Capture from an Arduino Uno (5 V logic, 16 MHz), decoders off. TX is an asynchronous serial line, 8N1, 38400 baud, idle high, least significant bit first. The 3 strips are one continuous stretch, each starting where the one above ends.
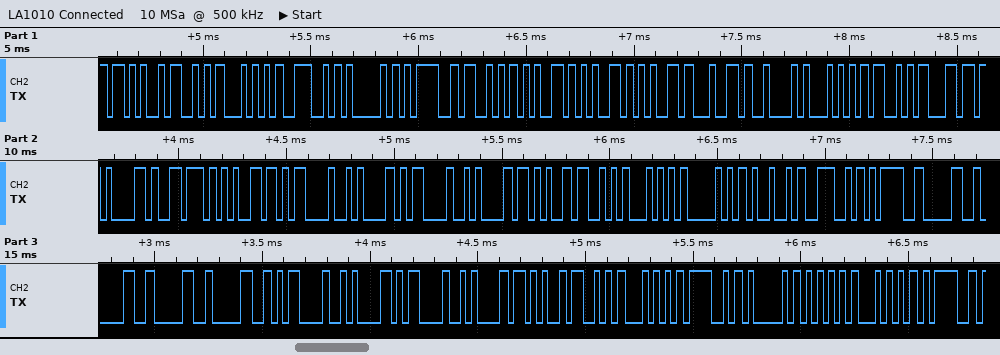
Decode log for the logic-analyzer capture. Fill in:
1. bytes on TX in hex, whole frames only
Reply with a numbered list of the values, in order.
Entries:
1. 0x2B 0x53 0x54 0x4E 0x41 0x3D 0x53 0x65 0x65 0x65 0x64 0x42 0x54 0x53 0x6C 0x61 0x76 0x65 0x0D 0x0A 0x0D 0x0A 0x2B 0x53 0x54 0x50 0x49 0x4E 0x3D 0x30 0x30 0x30 0x30 0x0D 0x0A 0x0D 0x0A 0x2B 0x53 0x54 0x4F 0x41 0x55 0x54 0x3D
